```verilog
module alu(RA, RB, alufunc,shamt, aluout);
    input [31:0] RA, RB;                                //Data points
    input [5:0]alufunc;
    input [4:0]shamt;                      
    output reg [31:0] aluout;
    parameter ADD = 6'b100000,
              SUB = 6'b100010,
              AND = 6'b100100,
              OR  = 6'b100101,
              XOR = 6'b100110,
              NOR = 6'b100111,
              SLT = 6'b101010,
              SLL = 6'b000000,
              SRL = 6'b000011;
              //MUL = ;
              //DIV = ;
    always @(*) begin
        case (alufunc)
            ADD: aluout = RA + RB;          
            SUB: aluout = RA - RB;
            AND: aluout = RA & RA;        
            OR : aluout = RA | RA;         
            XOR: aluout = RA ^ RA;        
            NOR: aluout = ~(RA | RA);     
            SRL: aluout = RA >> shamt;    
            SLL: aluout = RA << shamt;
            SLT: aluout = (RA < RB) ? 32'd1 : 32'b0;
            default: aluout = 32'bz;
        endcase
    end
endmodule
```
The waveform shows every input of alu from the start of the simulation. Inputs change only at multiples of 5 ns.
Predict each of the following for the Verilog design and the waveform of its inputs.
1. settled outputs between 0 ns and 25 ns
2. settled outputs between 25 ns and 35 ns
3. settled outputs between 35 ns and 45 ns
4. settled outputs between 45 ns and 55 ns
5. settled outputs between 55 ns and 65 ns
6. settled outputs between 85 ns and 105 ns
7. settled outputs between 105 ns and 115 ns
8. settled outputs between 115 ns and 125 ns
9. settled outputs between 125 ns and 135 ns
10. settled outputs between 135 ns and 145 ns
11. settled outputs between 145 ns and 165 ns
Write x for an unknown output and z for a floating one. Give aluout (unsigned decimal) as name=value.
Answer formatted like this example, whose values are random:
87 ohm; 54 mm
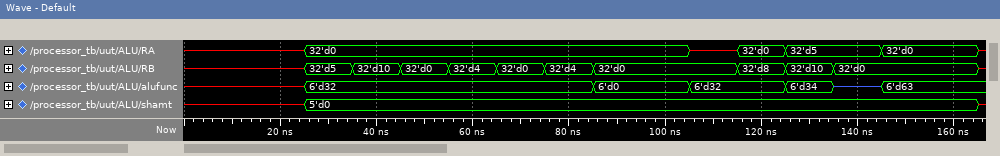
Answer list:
aluout=x; aluout=5; aluout=10; aluout=0; aluout=4; aluout=0; aluout=x; aluout=8; aluout=4294967291; aluout=z; aluout=z
